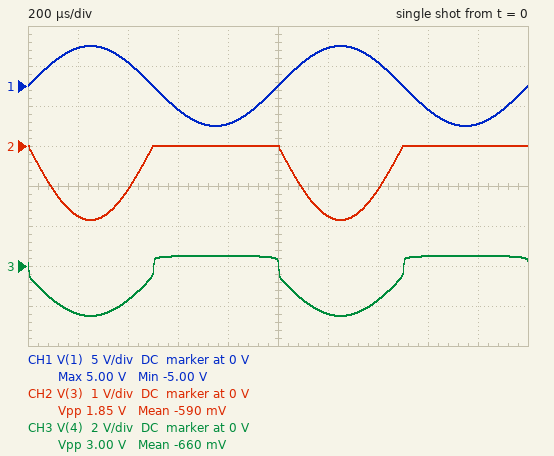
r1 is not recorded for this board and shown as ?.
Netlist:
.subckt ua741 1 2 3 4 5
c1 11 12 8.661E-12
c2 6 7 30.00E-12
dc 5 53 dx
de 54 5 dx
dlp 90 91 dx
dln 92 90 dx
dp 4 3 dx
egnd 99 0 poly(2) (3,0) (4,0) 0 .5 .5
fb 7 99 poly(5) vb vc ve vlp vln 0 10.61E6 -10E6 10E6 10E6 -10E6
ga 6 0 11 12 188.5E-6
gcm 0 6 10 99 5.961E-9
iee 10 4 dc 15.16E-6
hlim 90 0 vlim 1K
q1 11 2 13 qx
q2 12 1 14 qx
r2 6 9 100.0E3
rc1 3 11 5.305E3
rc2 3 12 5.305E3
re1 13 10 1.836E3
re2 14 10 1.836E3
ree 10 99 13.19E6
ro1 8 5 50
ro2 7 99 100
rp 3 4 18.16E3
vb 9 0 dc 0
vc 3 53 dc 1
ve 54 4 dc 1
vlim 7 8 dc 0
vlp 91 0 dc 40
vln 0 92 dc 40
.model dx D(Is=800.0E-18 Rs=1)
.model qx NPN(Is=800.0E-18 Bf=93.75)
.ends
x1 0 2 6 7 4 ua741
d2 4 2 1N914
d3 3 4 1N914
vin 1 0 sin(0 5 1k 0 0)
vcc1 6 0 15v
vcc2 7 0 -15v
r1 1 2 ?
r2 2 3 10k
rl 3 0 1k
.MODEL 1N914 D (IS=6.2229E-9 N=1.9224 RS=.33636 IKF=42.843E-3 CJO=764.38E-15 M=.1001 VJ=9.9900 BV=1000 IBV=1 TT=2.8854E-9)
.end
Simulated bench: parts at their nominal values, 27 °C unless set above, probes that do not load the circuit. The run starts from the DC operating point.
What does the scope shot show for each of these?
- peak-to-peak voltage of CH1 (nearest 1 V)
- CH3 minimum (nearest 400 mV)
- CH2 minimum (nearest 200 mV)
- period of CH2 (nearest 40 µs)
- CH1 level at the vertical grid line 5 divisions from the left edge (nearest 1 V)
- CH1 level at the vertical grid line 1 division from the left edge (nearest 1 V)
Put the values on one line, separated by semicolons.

10 V; -2.4 V; -1.8 V; 1.00 ms; 0 V; 5 V
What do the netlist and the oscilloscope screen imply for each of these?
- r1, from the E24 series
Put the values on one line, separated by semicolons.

27 kΩ
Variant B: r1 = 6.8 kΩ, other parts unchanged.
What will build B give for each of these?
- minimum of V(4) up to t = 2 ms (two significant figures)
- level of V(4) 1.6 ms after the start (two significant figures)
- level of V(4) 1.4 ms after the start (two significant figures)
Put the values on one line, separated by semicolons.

-8.1 V; 560 mV; -5.0 V
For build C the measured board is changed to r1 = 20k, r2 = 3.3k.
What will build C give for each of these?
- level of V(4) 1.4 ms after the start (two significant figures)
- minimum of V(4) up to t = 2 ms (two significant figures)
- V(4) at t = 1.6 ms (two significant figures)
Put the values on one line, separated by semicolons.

-1.1 V; -1.4 V; 500 mV
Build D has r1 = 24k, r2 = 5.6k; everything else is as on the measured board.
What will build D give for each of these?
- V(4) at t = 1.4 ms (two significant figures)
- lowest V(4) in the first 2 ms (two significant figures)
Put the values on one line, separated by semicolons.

-1.3 V; -1.8 V
